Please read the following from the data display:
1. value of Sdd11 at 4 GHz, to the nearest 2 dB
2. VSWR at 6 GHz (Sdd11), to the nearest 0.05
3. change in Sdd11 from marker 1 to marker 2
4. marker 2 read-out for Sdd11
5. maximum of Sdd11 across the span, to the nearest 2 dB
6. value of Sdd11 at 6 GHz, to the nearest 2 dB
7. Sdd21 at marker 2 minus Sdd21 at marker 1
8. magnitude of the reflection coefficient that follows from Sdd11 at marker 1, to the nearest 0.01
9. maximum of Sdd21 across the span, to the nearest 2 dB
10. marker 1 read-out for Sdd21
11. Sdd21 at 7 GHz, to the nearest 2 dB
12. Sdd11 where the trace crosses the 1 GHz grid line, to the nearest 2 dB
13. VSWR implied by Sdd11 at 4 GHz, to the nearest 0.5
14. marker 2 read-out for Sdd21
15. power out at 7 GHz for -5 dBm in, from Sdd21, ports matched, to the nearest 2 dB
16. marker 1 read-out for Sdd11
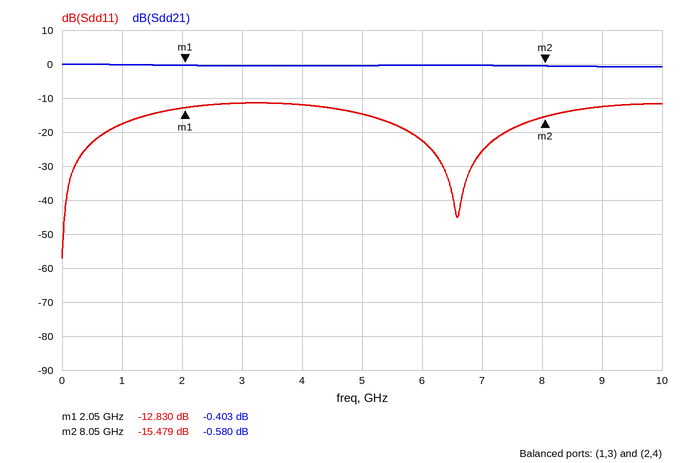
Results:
-12 dB
1.15
-2.649 dB
-15.479 dB
-12 dB
-22 dB
-0.177 dB
0.23
0 dB
-0.403 dB
0 dB
-18 dB
1.5
-0.580 dB
-6 dBm
-12.830 dB
